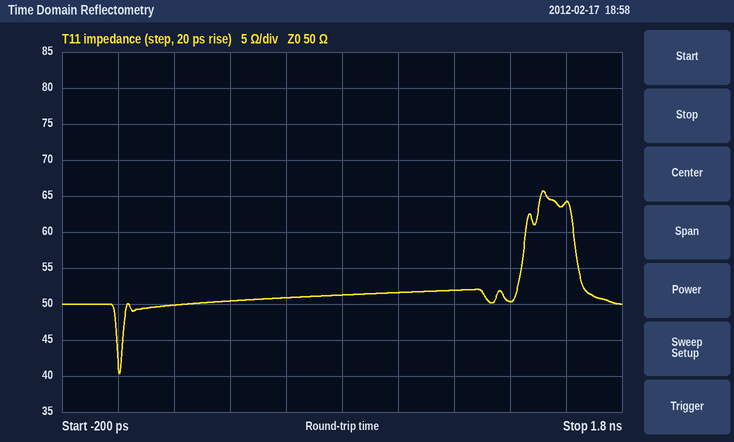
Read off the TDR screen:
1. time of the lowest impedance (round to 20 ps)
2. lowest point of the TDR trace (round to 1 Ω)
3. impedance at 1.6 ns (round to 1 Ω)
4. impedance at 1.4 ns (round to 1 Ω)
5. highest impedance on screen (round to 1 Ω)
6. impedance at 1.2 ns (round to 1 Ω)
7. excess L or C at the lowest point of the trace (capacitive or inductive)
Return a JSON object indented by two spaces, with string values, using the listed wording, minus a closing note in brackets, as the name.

{
  "time of the lowest impedance": "0 ps",
  "lowest point of the TDR trace": "40 Ω",
  "impedance at 1.6 ns": "64 Ω",
  "impedance at 1.4 ns": "50 Ω",
  "highest impedance on screen": "66 Ω",
  "impedance at 1.2 ns": "52 Ω",
  "excess L or C at the lowest point of the trace": "capacitive"
}
